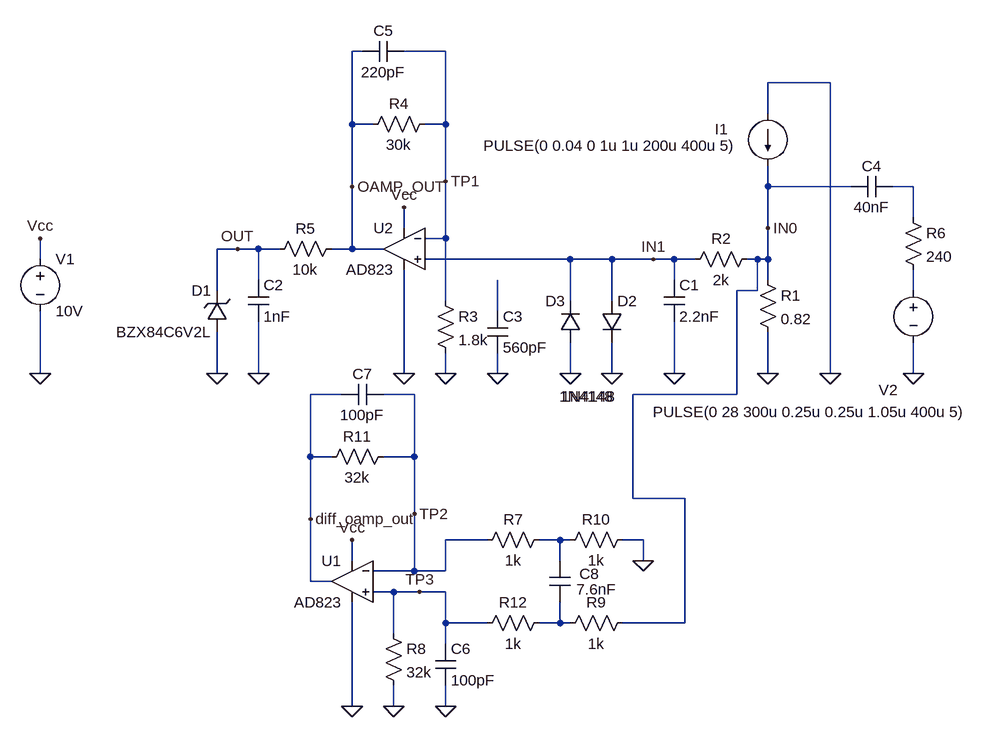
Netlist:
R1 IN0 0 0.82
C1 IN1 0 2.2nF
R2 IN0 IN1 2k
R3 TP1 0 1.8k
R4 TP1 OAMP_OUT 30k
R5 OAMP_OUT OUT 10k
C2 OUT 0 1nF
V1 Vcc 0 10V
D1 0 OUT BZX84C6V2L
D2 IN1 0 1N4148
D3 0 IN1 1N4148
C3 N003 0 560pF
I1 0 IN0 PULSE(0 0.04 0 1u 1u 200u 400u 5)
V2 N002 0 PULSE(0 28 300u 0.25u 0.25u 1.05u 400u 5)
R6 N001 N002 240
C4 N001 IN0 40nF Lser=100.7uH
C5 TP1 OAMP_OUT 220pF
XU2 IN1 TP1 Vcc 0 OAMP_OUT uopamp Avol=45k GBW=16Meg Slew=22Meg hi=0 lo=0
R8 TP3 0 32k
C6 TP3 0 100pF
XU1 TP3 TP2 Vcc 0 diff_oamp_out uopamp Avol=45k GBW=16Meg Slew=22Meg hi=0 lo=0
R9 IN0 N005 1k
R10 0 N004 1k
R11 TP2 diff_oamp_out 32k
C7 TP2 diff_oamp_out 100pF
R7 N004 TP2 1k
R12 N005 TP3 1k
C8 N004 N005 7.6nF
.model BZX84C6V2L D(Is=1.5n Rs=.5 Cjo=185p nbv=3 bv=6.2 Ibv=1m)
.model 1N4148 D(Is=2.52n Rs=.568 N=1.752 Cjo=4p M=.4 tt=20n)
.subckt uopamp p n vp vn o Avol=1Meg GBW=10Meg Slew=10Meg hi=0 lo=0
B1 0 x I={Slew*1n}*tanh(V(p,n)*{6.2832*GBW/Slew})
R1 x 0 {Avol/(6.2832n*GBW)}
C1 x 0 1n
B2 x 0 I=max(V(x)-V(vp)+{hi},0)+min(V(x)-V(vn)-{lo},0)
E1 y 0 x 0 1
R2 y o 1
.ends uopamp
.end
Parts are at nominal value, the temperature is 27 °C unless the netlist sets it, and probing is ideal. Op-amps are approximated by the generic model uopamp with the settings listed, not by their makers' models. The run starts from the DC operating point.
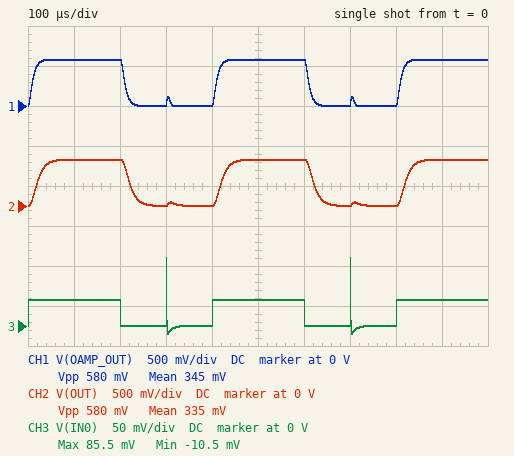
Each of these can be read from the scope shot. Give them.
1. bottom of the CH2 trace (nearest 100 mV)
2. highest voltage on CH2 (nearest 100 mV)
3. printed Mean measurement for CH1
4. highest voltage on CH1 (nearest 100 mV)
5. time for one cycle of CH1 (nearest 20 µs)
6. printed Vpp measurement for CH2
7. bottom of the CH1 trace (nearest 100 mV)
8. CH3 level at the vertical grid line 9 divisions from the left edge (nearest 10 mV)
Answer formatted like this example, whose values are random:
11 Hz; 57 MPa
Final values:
0 V; 600 mV; 345 mV; 600 mV; 400 µs; 580 mV; 0 V; 30 mV
